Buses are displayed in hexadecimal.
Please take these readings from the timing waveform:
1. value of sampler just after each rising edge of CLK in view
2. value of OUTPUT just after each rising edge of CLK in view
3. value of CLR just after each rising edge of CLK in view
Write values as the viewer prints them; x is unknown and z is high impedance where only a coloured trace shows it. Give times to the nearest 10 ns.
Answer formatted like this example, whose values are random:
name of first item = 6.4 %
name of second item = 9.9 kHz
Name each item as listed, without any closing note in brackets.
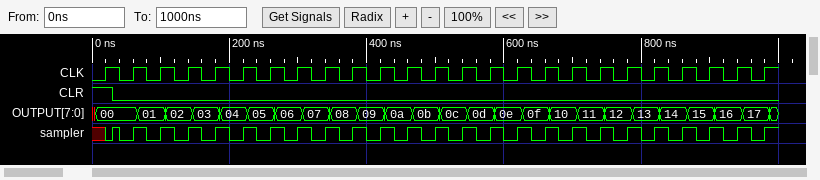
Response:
value of sampler just after each rising edge of CLK in view = 0 1 1 1 1 1 1 1 1 1 1 1 1 1 1 1 1 1 1 1 1 1 1 1 1
value of OUTPUT just after each rising edge of CLK in view = 00, 00, 01, 02, 03, 04, 05, 06, 07, 08, 09, 0a, 0b, 0c, 0d, 0e, 0f, 10, 11, 12, 13, 14, 15, 16, 17
value of CLR just after each rising edge of CLK in view = 1 0 0 0 0 0 0 0 0 0 0 0 0 0 0 0 0 0 0 0 0 0 0 0 0
